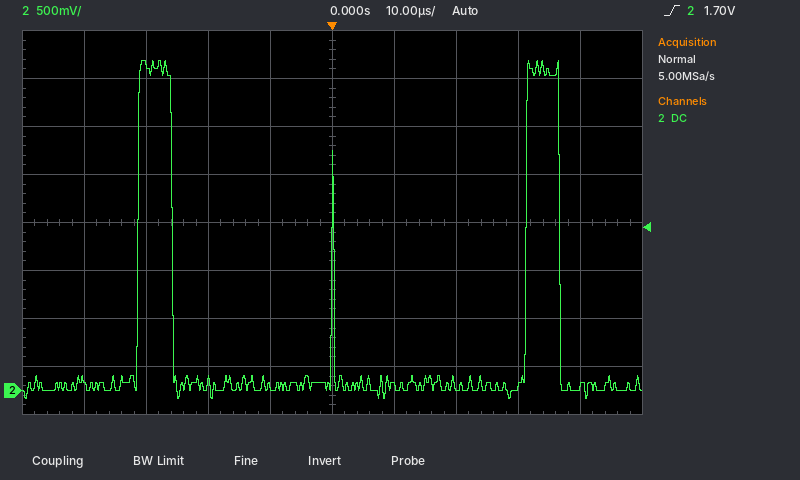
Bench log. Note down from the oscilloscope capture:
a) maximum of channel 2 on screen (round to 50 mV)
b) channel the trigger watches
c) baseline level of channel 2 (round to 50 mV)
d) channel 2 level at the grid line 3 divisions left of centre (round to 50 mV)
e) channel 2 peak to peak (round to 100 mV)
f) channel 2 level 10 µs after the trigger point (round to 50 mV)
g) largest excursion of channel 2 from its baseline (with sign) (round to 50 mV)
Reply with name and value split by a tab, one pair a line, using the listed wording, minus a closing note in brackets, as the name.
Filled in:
maximum of channel 2 on screen	3.45 V
channel the trigger watches	channel 2
baseline level of channel 2	50 mV
channel 2 level at the grid line 3 divisions left of centre	3.40 V
channel 2 peak to peak	3.50 V
channel 2 level 10 µs after the trigger point	50 mV
largest excursion of channel 2 from its baseline (with sign)	+3.40 V
